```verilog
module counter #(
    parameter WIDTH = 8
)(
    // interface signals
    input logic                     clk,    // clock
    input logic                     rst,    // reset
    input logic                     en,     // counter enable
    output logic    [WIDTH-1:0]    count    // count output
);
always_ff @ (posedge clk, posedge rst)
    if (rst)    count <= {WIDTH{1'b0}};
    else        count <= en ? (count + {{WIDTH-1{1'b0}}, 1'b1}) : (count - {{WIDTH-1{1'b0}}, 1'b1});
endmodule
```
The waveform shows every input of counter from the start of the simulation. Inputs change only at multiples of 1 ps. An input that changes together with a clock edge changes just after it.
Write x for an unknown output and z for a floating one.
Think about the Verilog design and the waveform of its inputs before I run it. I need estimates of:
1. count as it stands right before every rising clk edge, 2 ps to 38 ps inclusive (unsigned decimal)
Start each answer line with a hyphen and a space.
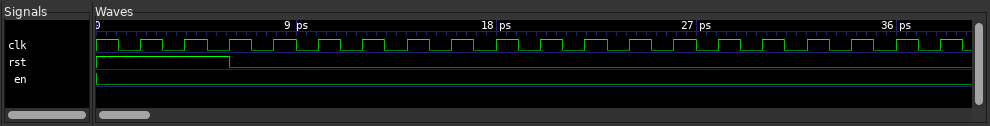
- 0, 0, 0, 0, 255, 254, 253, 252, 251, 250, 249, 248, 247, 246, 245, 244, 243, 242, 241
